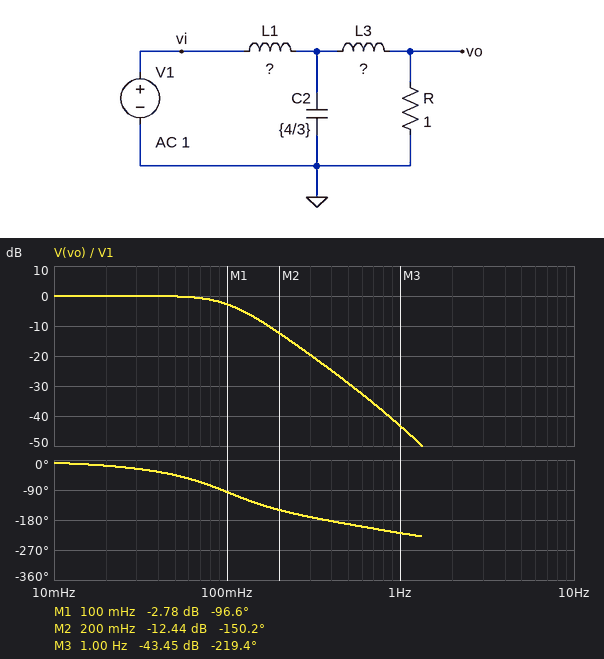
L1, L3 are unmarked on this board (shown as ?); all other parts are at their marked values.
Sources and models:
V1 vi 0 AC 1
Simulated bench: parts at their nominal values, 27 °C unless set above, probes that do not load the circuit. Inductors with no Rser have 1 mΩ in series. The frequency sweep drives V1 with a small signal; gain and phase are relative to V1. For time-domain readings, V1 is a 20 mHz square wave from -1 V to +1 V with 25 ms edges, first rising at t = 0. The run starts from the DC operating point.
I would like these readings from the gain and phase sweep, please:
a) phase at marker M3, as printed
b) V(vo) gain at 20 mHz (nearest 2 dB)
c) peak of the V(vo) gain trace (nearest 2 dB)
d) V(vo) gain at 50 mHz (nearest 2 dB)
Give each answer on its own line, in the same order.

-219.4 deg
0 dB
0 dB
0 dB
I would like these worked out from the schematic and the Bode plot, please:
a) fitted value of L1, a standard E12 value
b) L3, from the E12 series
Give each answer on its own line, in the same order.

2.2 H
150 mH
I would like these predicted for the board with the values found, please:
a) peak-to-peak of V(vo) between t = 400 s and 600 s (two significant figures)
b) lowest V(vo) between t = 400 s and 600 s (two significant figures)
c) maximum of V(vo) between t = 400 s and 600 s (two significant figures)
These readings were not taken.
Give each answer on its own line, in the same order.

2.2 V
-1.1 V
1.1 V
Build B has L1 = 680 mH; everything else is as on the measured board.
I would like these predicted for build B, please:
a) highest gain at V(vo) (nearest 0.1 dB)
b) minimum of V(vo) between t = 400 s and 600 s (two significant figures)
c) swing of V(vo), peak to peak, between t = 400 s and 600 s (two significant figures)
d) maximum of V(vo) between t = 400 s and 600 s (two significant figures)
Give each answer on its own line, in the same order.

3.1 dB
-1.6 V
3.1 V
1.6 V
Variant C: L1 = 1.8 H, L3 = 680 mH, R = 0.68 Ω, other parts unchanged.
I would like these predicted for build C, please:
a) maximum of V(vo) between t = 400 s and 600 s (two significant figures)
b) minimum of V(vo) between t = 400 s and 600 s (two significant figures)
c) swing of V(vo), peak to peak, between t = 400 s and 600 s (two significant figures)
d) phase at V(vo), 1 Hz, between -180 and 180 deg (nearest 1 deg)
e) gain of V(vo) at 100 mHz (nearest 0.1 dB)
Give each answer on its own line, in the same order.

1.0 V
-1.0 V
2.0 V
99 deg
-4.6 dB
